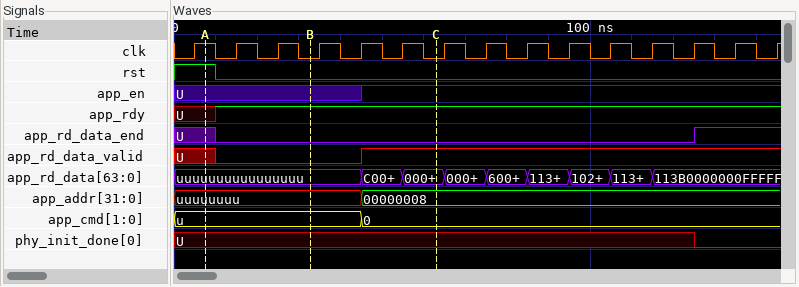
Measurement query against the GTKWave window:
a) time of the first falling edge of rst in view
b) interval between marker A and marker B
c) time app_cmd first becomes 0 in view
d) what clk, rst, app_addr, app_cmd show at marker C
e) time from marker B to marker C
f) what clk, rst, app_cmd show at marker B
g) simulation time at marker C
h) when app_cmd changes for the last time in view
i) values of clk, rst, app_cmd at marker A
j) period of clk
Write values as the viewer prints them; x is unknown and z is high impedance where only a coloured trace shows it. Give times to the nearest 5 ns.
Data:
10 ns
25 ns
45 ns
clk=0, rst=0, app_addr=00000008, app_cmd=0
30 ns
clk=0, rst=0, app_cmd=u
65 ns
45 ns
clk=1, rst=1, app_cmd=u
10 ns
